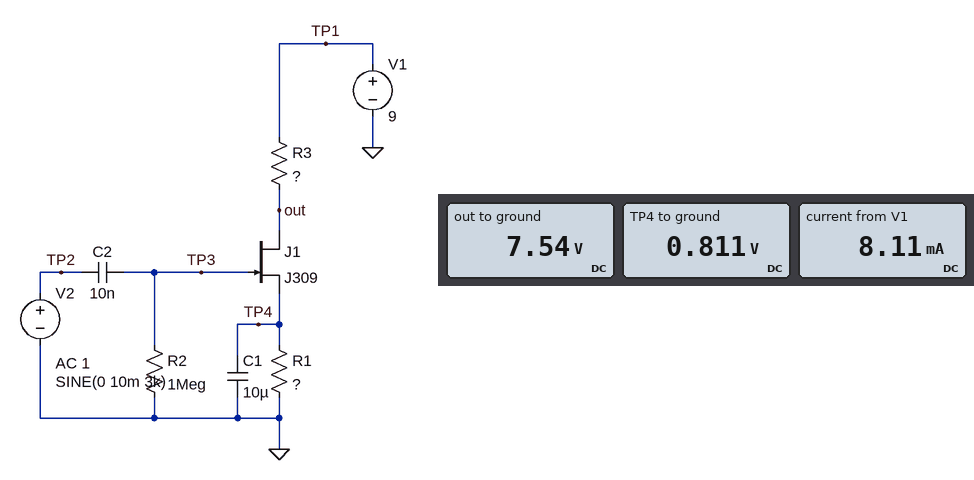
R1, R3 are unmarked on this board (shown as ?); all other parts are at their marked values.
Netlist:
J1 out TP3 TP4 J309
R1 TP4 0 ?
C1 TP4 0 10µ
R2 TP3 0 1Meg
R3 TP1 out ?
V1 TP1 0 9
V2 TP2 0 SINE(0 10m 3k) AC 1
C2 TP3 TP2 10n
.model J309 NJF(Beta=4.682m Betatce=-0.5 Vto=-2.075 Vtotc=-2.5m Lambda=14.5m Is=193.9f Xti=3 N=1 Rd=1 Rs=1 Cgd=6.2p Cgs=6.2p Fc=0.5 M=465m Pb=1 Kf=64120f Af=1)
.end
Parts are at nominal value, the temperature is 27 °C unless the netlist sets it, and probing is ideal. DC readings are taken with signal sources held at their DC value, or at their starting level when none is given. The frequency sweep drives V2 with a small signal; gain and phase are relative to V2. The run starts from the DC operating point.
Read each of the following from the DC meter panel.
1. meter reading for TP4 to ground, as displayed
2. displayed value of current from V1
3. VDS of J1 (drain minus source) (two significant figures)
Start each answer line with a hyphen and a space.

- 0.811 V
- 8.11 mA
- 6.7 V
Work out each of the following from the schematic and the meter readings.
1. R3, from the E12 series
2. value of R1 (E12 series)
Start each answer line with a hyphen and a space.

- 180 Ω
- 100 Ω
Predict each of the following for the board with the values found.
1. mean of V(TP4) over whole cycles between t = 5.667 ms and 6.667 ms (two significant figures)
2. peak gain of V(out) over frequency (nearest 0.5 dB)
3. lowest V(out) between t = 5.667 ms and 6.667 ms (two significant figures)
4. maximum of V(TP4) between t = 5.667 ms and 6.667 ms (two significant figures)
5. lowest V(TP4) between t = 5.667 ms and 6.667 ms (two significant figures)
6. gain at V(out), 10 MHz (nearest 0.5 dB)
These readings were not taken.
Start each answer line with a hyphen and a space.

- 810 mV
- 7.0 dB
- 7.5 V
- 810 mV
- 810 mV
- 7.0 dB
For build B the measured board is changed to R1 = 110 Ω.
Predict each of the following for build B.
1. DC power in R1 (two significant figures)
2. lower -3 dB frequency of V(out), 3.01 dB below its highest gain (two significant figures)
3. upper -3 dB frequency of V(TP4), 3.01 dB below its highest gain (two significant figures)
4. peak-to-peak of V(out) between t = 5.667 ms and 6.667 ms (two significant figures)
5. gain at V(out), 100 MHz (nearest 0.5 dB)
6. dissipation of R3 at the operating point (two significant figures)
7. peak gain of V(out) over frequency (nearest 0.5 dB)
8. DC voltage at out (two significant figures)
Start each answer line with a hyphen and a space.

- 6.5 mW
- 270 Hz
- 370 Hz
- 44 mV
- 6.5 dB
- 11 mW
- 7.0 dB
- 7.6 V
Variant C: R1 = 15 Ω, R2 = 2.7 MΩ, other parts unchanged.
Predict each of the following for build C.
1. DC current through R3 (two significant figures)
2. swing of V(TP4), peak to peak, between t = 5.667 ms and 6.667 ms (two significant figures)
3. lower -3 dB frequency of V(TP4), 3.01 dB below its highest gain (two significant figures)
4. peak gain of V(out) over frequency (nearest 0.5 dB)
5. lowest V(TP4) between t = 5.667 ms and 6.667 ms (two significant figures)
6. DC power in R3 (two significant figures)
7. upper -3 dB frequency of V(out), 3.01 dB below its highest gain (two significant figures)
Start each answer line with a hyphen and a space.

- 17 mA
- 1.7 mV
- 5.8 Hz
- 10.0 dB
- 250 mV
- 50 mW
- 440 MHz
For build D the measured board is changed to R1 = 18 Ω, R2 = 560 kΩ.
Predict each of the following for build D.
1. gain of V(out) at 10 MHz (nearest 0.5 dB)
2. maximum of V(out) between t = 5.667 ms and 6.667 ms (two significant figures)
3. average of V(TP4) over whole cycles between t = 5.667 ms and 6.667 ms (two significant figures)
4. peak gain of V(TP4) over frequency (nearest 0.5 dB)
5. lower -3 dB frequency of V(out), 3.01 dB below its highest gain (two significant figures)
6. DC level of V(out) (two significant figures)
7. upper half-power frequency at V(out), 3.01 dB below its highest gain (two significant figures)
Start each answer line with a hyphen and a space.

- 9.5 dB
- 6.2 V
- 290 mV
- -13.0 dB
- 69 Hz
- 6.1 V
- 450 MHz
